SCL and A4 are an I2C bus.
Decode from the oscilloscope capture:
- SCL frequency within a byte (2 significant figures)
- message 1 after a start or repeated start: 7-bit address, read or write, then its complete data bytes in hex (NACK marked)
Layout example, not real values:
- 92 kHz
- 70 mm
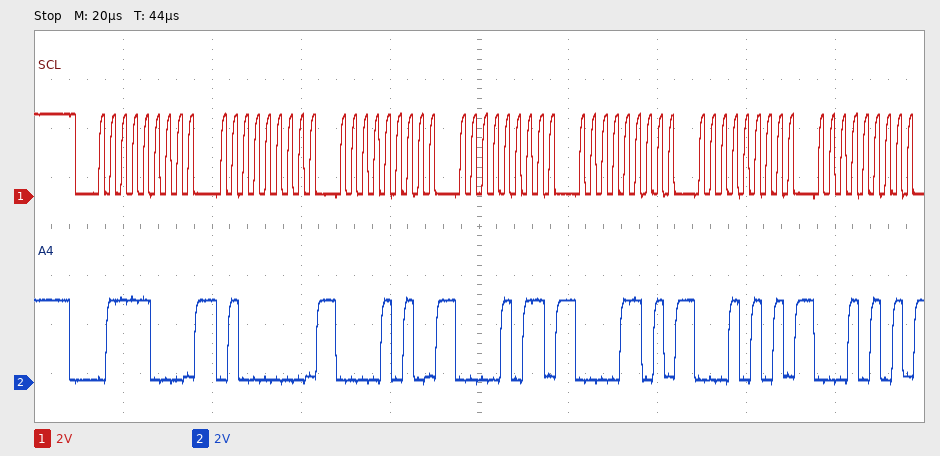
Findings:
- 400 kHz
- 0x3C write: 40 0A 0B 0D 15 15
